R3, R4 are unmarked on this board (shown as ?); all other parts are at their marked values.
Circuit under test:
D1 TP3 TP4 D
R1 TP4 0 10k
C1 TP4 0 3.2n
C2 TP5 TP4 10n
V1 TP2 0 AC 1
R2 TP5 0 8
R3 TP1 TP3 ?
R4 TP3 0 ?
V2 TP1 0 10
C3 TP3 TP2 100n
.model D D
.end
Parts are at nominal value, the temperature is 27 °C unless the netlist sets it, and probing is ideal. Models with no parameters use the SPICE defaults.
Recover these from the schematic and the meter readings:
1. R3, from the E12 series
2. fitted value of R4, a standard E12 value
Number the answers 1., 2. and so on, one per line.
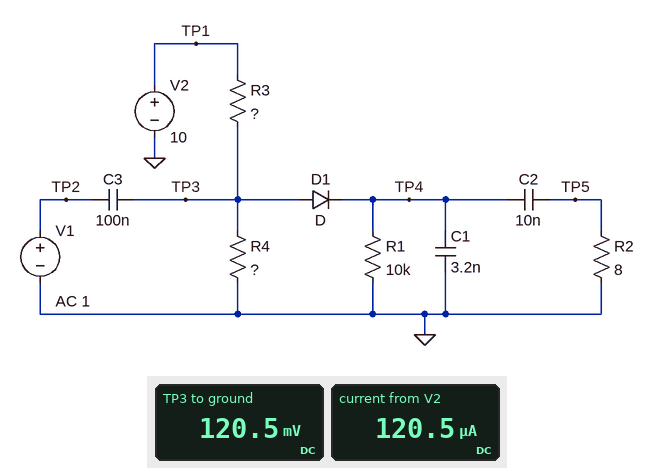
1. 82 kΩ
2. 1 kΩ
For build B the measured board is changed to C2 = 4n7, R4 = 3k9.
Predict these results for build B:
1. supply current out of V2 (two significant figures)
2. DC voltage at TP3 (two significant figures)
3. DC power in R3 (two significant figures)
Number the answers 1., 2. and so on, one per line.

1. 120 µA
2. 450 mV
3. 1.1 mW
